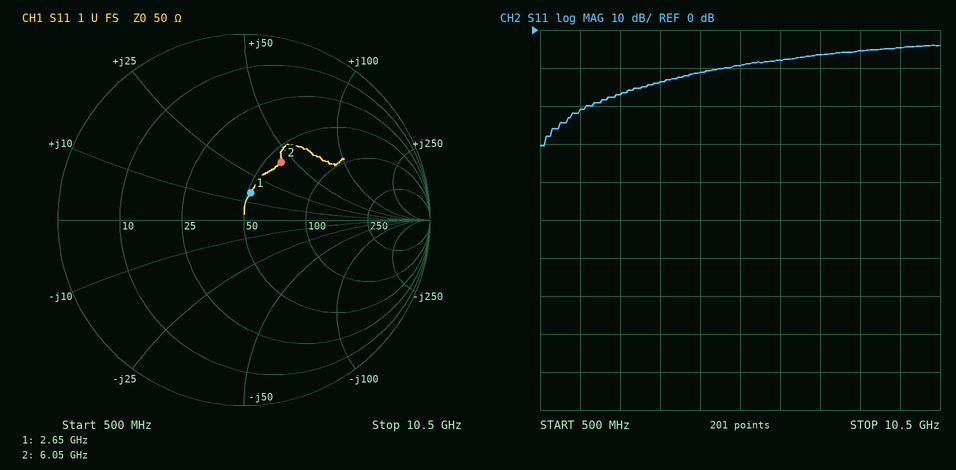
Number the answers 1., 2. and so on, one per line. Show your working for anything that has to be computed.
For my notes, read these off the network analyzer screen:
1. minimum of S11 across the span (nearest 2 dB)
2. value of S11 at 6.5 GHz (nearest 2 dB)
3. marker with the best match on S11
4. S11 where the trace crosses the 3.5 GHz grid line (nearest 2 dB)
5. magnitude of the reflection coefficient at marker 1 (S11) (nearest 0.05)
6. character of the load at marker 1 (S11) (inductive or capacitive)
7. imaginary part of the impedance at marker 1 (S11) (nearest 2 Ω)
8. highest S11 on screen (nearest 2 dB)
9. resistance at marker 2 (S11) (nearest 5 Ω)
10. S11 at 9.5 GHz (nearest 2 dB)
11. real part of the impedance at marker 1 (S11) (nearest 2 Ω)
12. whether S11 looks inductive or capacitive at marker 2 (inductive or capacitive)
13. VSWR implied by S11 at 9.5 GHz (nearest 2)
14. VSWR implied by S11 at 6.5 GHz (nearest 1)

1. -30 dB
2. -8 dB
3. marker 1
4. -14 dB
5. 0.15
6. inductive
7. +16 Ω
8. -4 dB
9. 60 Ω
10. -4 dB
11. 52 Ω
12. inductive
13. |Γ| = 10^(-4/20) = 0.6310; VSWR = (1 + 0.6310)/(1 − 0.6310) ≈ 4
14. |Γ| = 10^(-8/20) = 0.3981; VSWR = (1 + 0.3981)/(1 − 0.3981) ≈ 2
